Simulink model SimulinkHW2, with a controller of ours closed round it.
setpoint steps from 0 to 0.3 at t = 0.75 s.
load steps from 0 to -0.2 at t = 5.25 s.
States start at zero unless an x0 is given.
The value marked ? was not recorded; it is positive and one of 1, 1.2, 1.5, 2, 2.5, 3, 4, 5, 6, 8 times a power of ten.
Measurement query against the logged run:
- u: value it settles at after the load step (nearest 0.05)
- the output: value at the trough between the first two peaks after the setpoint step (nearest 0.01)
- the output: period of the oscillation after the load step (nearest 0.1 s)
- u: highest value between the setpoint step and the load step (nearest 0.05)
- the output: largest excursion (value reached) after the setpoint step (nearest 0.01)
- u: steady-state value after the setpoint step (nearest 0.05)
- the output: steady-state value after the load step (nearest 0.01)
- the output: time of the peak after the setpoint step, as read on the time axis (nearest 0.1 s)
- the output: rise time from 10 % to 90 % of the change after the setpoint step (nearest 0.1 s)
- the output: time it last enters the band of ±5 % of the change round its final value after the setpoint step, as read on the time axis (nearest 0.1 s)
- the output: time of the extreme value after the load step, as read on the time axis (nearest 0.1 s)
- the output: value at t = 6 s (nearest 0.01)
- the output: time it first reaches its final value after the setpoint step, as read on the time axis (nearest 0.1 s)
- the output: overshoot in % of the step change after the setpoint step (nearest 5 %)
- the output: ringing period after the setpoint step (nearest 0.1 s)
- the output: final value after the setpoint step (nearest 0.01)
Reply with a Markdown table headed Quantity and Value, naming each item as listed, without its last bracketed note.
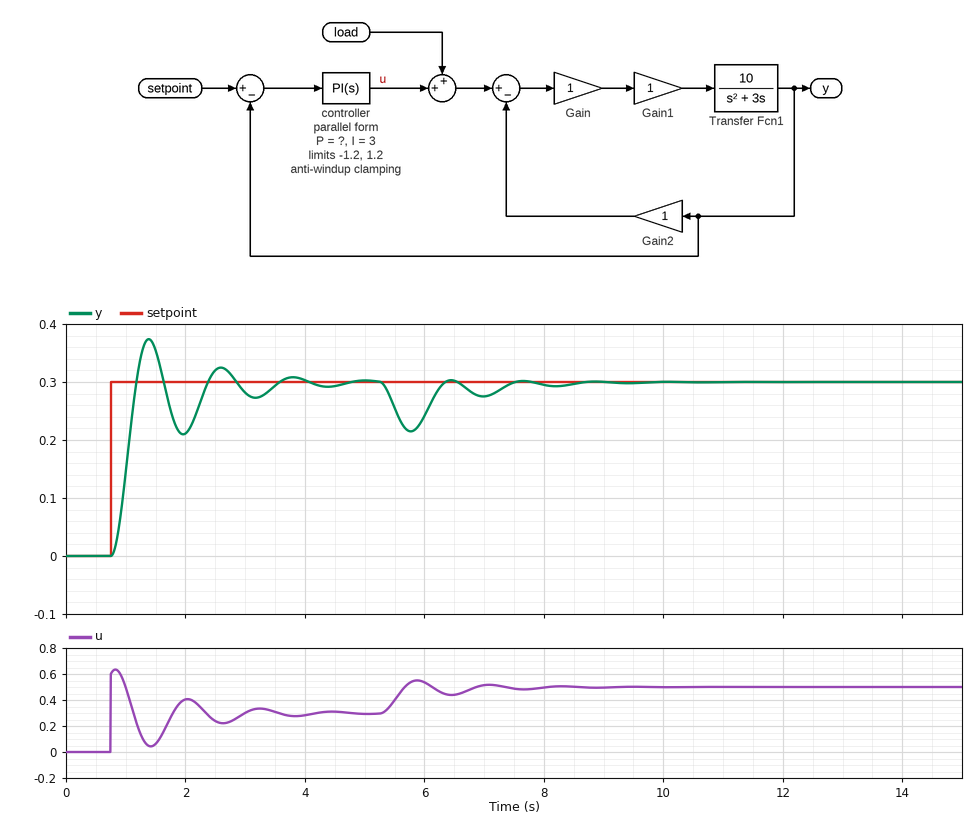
| Quantity | Value |
|---|---|
| u: value it settles at after the load step | 0.50 |
| the output: value at the trough between the first two peaks after the setpoint step | 0.21 |
| the output: period of the oscillation after the load step | 1.2 s |
| u: highest value between the setpoint step and the load step | 0.65 |
| the output: largest excursion (value reached) after the setpoint step | 0.37 |
| u: steady-state value after the setpoint step | 0.30 |
| the output: steady-state value after the load step | 0.30 |
| the output: time of the peak after the setpoint step, as read on the time axis | 1.4 s |
| the output: rise time from 10 % to 90 % of the change after the setpoint step | 0.3 s |
| the output: time it last enters the band of ±5 % of the change round its final value after the setpoint step, as read on the time axis | 3.4 s |
| the output: time of the extreme value after the load step, as read on the time axis | 5.8 s |
| the output: value at t = 6 s | 0.24 |
| the output: time it first reaches its final value after the setpoint step, as read on the time axis | 1.2 s |
| the output: overshoot in % of the step change after the setpoint step | 25 % |
| the output: ringing period after the setpoint step | 1.2 s |
| the output: final value after the setpoint step | 0.30 |
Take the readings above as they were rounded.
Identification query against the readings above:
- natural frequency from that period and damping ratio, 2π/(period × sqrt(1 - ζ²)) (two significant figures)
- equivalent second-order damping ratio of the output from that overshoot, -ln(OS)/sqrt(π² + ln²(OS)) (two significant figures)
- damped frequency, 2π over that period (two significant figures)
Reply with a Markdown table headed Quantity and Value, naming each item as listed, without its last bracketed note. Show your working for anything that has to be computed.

| Quantity | Value |
|---|---|
| natural frequency from that period and damping ratio, 2π/(period × sqrt(1 - ζ²)) | 2π / (1.2 × sqrt(1 - 0.4²)) = 5.7 rad/s |
| equivalent second-order damping ratio of the output from that overshoot, -ln(OS)/sqrt(π² + ln²(OS)) | ln(0.25) = -1.386; 1.386 / sqrt(9.870 + 1.922) = 0.40 |
| damped frequency, 2π over that period | 2π / 1.2 = 5.2 rad/s |
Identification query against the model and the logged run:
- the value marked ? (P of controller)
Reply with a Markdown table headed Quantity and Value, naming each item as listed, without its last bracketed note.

| Quantity | Value |
|---|---|
| the value marked ? | 2 |
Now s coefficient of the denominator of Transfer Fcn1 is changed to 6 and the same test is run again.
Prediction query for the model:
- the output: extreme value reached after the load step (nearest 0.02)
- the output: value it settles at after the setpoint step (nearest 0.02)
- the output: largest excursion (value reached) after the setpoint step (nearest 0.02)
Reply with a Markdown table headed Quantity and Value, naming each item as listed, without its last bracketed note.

| Quantity | Value |
|---|---|
| the output: extreme value reached after the load step | 0.24 |
| the output: value it settles at after the setpoint step | 0.30 |
| the output: largest excursion (value reached) after the setpoint step | 0.32 |
